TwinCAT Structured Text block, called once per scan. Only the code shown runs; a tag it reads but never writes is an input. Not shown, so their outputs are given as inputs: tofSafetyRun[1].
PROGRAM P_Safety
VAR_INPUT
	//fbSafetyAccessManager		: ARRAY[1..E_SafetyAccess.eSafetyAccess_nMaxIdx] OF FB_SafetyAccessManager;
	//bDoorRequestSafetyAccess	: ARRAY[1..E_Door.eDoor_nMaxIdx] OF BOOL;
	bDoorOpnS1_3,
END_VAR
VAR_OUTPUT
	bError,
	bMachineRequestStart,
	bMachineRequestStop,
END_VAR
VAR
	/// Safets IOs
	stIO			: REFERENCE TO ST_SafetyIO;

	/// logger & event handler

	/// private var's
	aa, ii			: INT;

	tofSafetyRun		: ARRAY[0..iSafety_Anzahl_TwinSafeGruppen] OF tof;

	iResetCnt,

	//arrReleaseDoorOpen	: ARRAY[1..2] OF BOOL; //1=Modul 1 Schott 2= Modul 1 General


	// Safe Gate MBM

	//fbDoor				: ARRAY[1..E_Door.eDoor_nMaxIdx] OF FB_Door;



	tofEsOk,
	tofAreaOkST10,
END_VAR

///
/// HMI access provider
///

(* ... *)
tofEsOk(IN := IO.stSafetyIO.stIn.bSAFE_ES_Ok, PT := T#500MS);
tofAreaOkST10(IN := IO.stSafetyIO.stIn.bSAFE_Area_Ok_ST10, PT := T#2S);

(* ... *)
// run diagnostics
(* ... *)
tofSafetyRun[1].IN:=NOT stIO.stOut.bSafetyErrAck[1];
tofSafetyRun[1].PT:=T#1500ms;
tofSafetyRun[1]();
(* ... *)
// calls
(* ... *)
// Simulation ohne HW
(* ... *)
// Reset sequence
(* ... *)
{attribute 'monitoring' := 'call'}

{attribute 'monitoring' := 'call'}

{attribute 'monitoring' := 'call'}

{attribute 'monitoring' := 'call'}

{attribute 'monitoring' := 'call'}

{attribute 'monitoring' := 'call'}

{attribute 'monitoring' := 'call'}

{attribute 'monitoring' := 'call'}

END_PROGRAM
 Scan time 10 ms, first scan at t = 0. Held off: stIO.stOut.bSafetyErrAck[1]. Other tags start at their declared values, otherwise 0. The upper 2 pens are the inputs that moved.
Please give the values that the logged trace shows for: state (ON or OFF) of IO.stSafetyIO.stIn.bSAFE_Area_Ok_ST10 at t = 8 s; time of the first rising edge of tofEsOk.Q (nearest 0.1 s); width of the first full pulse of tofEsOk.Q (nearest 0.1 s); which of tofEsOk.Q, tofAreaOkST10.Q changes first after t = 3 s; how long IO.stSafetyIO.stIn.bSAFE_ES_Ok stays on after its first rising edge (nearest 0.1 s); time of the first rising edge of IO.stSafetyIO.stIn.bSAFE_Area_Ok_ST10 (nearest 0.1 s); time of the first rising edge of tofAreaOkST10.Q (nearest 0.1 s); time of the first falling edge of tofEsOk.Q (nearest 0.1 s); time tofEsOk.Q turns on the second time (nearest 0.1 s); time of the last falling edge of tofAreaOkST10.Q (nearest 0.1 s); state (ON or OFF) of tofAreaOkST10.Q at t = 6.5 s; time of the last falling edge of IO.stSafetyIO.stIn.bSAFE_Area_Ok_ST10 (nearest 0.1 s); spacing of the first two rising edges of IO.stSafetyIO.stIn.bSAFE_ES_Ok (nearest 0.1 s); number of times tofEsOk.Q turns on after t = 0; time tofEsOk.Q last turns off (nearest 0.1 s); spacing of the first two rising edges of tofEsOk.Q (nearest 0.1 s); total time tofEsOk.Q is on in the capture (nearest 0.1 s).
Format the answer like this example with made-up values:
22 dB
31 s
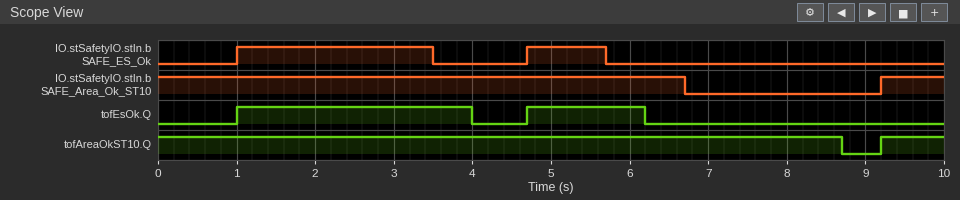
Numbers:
OFF
1.0 s
3.0 s
tofEsOk.Q
2.5 s
9.2 s
9.2 s
4.0 s
4.7 s
8.7 s
ON
6.7 s
3.7 s
2
6.2 s
3.7 s
4.5 s
